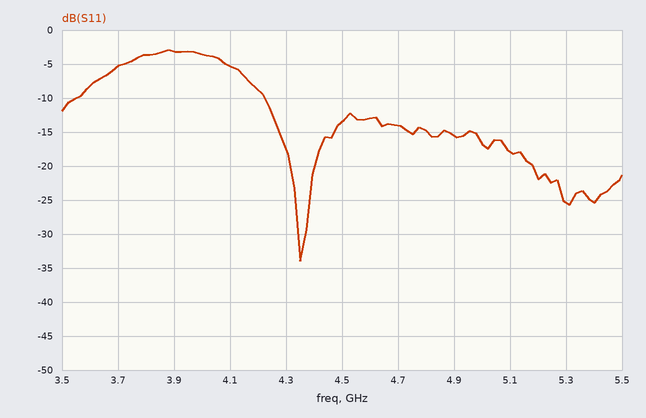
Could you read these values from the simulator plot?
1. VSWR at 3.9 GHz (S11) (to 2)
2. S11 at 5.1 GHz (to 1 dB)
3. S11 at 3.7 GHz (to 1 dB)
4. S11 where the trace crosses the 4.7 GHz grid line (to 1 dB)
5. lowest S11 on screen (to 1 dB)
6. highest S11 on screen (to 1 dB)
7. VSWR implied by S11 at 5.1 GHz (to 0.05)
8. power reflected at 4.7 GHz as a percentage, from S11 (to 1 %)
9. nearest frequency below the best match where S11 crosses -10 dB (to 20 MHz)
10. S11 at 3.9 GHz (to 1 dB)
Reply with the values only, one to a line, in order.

6
-18 dB
-5 dB
-14 dB
-34 dB
-3 dB
1.30
4 %
4.22 GHz
-3 dB
